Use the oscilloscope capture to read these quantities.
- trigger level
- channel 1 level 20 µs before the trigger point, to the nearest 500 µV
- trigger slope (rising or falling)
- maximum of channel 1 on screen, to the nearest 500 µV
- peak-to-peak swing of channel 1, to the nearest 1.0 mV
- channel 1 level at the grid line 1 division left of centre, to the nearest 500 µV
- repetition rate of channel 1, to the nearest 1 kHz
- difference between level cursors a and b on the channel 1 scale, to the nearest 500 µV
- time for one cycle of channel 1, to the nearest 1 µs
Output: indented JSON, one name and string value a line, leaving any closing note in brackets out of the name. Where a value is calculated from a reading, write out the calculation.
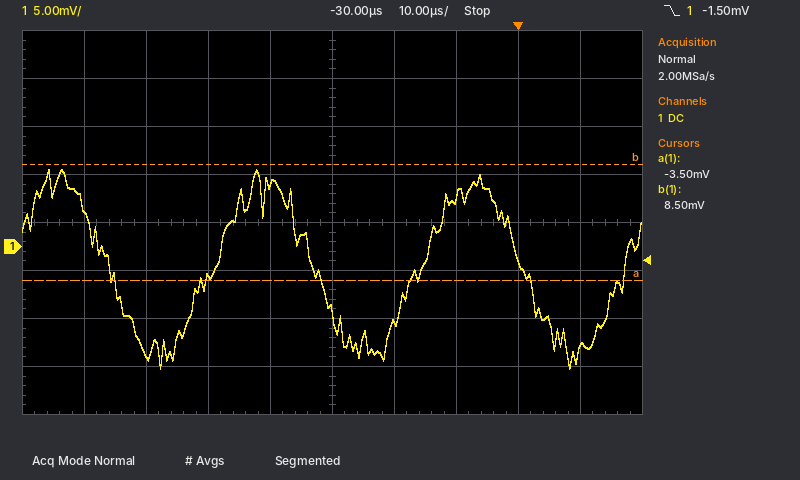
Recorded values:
{
  "trigger level": "-1.50 mV",
  "channel 1 level 20 µs before the trigger point, to the nearest 500 µV": "-8.0 mV",
  "trigger slope": "falling",
  "maximum of channel 1 on screen, to the nearest 500 µV": "8.0 mV",
  "peak-to-peak swing of channel 1, to the nearest 1.0 mV": "21.0 mV",
  "channel 1 level at the grid line 1 division left of centre, to the nearest 500 µV": "6.5 mV",
  "repetition rate of channel 1, to the nearest 1 kHz": "1 / 33 µs ≈ 30 kHz",
  "difference between level cursors a and b on the channel 1 scale, to the nearest 500 µV": "12.0 mV",
  "time for one cycle of channel 1, to the nearest 1 µs": "33 µs"
}
